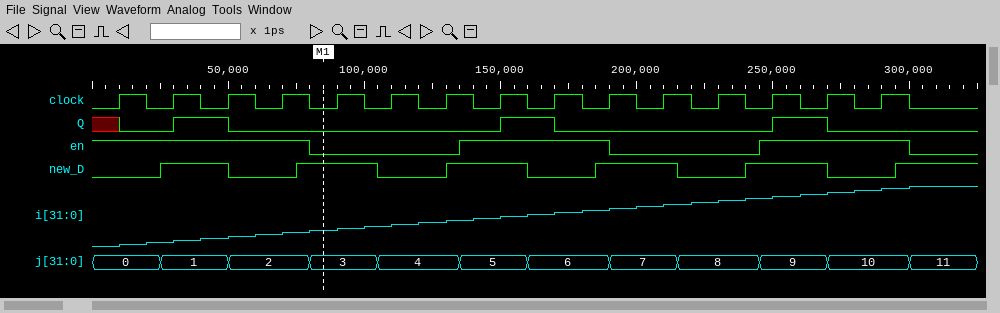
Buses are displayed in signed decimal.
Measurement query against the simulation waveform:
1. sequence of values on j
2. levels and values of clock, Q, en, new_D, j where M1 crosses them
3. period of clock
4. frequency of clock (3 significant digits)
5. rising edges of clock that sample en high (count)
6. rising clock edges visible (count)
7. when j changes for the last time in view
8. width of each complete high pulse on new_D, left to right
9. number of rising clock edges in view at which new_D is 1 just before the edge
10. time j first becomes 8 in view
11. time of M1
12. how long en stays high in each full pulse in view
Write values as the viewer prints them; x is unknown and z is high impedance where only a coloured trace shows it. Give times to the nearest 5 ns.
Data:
0, 1, 2, 3, 4, 5, 6, 7, 8, 9, 10, 11
clock=0, Q=0, en=0, new_D=1, j=3
20 ns
50.0 MHz
10
15
300 ns
25 ns, 30 ns, 30 ns, 30 ns, 30 ns
8
215 ns
85 ns
55 ns, 55 ns
